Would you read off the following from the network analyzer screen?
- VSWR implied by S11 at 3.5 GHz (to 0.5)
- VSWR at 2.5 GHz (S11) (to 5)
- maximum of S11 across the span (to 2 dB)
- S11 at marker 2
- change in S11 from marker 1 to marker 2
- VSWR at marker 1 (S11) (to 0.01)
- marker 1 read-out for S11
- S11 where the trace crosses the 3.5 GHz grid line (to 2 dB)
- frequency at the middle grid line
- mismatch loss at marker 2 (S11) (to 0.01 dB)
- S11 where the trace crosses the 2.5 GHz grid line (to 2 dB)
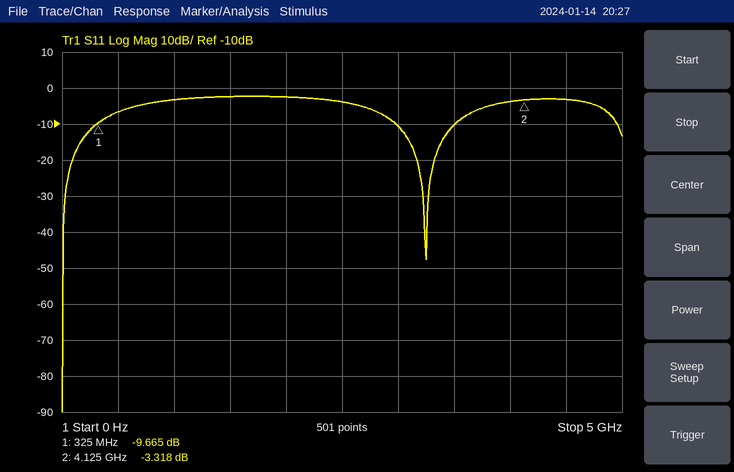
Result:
2.0
5
-2 dB
-3.318 dB
6.347 dB
1.98
-9.665 dB
-10 dB
2.5 GHz
2.72 dB
-4 dB
